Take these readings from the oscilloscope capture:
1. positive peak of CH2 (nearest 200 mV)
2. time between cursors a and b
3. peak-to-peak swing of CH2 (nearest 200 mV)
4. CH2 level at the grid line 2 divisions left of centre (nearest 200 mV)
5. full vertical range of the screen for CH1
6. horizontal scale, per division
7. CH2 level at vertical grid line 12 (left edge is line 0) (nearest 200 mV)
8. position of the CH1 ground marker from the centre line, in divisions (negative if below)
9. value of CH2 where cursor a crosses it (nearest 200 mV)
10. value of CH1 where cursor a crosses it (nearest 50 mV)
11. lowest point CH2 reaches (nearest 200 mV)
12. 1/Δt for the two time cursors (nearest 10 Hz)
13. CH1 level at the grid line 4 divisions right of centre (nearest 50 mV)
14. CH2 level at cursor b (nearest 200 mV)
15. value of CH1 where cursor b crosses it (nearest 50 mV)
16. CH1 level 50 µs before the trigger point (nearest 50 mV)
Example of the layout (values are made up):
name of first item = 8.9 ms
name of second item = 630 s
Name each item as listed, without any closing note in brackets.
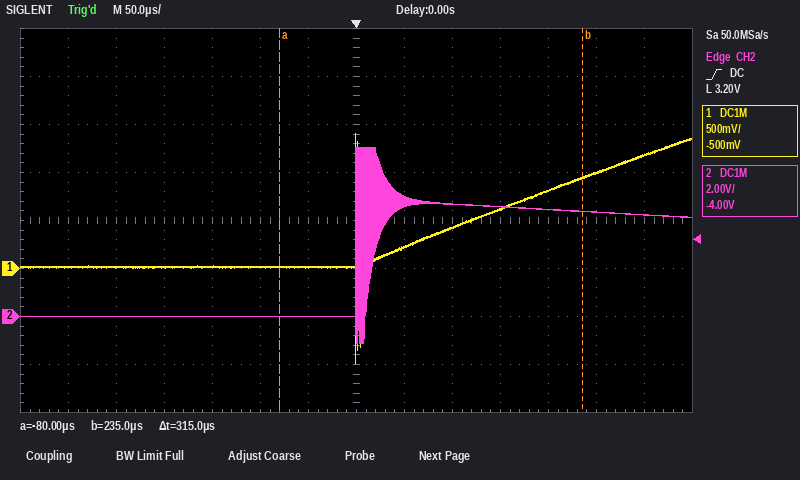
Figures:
positive peak of CH2 = 7.0 V
time between cursors a and b = 315 µs
peak-to-peak swing of CH2 = 8.2 V
CH2 level at the grid line 2 divisions left of centre = 0.0 V
full vertical range of the screen for CH1 = 4 V
horizontal scale, per division = 50 µs
CH2 level at vertical grid line 12 (left edge is line 0) = 4.4 V
position of the CH1 ground marker from the centre line, in divisions = -1.0 div
value of CH2 where cursor a crosses it = 0.0 V
value of CH1 where cursor a crosses it = 0 mV
lowest point CH2 reaches = -1.2 V
1/Δt for the two time cursors = 3.17 kHz
CH1 level at the grid line 4 divisions right of centre = 800 mV
CH2 level at cursor b = 4.4 V
value of CH1 where cursor b crosses it = 950 mV
CH1 level 50 µs before the trigger point = 0 mV
